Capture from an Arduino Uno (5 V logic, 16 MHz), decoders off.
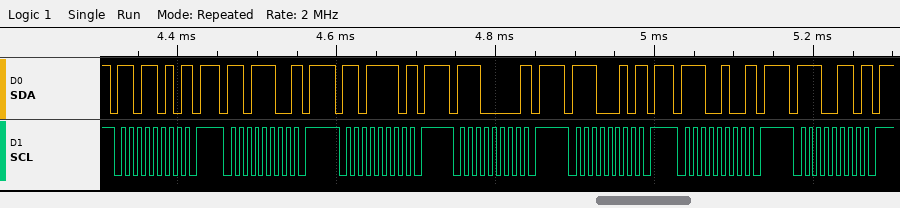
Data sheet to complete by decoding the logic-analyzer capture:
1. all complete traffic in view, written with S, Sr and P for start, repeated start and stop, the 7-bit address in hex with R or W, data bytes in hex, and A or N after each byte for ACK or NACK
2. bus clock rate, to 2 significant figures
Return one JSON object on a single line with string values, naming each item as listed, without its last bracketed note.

{"all complete traffic in view, written with S, Sr and P for start, repeated start and stop, the 7-bit address in hex with R or W, data bytes in hex, and A or N after each byte for ACK or NACK": "S 6DW N P S 6EW N P S 6FW N P S 70W N P S 71W N P S 72W N P S 73W N P", "bus clock rate, to 2 significant figures": "100 kHz"}
